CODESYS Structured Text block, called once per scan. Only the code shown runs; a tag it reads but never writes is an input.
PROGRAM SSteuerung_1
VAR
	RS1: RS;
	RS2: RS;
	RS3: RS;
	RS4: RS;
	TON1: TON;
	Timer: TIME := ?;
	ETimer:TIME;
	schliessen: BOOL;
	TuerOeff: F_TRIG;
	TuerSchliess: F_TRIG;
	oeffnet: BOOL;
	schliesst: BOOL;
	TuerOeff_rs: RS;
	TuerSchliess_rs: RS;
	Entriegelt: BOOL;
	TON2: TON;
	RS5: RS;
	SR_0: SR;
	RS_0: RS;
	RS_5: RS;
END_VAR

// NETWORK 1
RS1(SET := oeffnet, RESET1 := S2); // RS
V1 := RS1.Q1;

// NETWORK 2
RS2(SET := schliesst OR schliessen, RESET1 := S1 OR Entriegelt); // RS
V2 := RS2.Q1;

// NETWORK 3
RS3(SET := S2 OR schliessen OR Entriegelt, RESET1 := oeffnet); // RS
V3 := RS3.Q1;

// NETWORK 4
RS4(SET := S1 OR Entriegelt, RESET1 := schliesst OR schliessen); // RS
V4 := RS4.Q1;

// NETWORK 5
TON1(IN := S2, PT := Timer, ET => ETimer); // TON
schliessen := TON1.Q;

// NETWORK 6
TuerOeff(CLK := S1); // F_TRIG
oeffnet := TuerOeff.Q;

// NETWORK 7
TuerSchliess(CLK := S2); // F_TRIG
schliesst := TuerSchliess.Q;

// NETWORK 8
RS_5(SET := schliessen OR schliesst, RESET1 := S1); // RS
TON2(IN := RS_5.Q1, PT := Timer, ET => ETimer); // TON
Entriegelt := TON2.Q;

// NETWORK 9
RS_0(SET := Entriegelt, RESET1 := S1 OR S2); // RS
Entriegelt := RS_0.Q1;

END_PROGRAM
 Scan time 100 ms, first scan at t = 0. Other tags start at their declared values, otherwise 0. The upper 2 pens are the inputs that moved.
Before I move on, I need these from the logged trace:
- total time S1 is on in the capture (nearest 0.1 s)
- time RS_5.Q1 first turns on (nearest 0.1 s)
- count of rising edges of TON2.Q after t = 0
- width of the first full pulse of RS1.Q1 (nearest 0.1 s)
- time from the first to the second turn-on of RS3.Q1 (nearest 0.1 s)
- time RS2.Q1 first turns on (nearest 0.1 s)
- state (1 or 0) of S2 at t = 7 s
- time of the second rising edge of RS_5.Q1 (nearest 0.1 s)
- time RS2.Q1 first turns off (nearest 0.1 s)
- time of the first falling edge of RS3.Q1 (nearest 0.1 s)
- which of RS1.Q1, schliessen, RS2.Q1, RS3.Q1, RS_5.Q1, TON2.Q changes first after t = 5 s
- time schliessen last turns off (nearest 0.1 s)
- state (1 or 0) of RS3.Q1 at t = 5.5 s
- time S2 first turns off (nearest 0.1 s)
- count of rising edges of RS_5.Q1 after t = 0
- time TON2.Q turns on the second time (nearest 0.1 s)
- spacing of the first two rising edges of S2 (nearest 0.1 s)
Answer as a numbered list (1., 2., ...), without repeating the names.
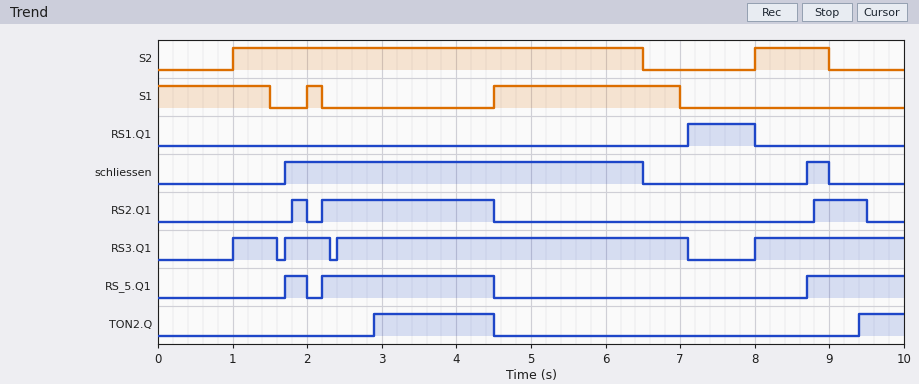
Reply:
1. 4.2 s
2. 1.7 s
3. 2
4. 0.9 s
5. 0.7 s
6. 1.8 s
7. 0
8. 2.2 s
9. 2.0 s
10. 1.6 s
11. schliessen
12. 9.0 s
13. 1
14. 6.5 s
15. 3
16. 9.4 s
17. 7.0 s
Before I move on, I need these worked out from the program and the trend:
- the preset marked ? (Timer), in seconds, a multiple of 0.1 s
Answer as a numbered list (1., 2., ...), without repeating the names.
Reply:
1. 0.7 s
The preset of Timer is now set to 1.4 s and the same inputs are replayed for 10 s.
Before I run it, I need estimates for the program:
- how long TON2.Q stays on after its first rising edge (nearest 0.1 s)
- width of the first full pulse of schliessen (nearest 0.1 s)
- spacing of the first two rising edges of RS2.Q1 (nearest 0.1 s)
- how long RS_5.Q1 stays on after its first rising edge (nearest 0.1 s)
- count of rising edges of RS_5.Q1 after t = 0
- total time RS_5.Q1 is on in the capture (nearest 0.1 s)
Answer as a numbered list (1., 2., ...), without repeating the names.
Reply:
1. 0.7 s
2. 4.1 s
3. 6.6 s
4. 2.1 s
5. 2
6. 3.1 s
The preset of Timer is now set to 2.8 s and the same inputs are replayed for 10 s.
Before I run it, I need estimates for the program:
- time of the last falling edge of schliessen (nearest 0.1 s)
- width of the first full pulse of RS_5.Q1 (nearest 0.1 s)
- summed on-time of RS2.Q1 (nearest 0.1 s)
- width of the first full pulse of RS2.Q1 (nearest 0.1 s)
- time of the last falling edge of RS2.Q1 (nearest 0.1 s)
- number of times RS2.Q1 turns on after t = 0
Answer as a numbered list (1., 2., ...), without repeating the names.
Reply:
1. 6.5 s
2. 0.7 s
3. 1.5 s
4. 0.6 s
5. 4.5 s
6. 2
